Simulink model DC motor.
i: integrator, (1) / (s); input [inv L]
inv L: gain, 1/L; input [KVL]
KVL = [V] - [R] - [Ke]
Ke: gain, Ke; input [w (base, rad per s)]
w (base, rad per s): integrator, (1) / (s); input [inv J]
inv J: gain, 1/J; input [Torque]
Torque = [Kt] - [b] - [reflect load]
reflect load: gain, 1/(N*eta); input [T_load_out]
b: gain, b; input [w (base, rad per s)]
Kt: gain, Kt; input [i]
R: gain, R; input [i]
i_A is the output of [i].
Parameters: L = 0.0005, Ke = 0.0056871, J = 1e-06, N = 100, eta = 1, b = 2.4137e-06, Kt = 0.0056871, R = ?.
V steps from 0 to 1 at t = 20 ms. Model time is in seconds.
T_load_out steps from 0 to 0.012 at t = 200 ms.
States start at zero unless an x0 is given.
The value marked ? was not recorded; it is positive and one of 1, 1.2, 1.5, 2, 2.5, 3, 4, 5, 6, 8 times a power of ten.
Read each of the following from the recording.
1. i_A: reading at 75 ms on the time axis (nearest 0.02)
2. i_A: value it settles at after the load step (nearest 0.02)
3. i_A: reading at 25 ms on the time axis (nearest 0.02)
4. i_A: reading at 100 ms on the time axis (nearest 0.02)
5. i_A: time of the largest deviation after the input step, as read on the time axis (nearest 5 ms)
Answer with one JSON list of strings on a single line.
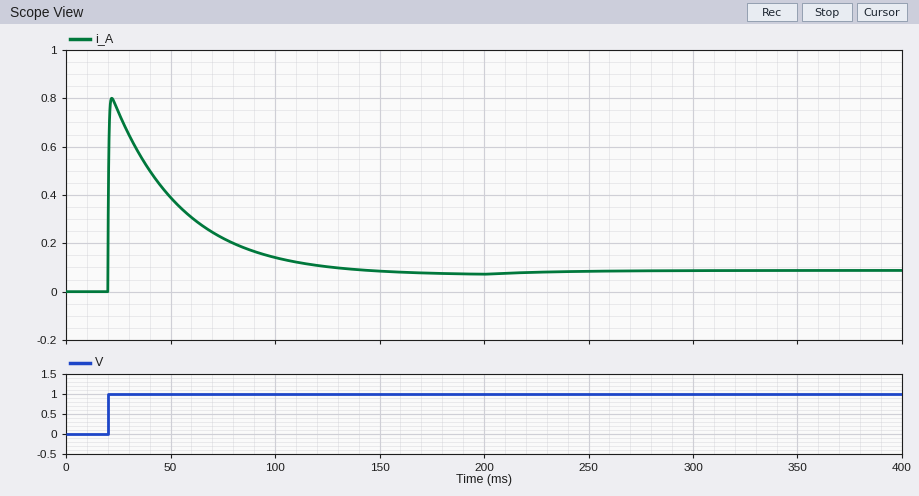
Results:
["0.22", "0.08", "0.74", "0.14", "20 ms"]
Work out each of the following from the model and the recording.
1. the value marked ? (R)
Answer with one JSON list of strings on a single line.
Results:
["1.2"]
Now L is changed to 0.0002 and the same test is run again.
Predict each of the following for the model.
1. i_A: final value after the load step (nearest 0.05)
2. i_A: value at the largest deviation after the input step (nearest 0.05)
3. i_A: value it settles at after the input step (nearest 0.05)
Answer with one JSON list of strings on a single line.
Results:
["0.10", "0.80", "0.05"]
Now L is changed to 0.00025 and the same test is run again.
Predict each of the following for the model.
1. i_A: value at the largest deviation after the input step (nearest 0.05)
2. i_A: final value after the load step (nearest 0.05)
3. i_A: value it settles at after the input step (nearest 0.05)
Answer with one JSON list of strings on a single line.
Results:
["0.80", "0.10", "0.05"]
